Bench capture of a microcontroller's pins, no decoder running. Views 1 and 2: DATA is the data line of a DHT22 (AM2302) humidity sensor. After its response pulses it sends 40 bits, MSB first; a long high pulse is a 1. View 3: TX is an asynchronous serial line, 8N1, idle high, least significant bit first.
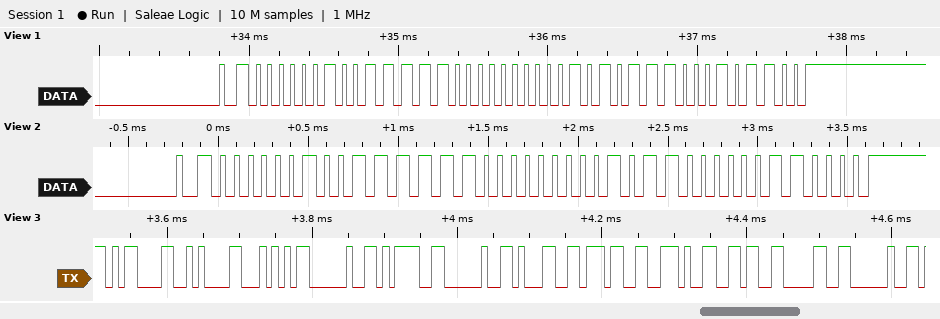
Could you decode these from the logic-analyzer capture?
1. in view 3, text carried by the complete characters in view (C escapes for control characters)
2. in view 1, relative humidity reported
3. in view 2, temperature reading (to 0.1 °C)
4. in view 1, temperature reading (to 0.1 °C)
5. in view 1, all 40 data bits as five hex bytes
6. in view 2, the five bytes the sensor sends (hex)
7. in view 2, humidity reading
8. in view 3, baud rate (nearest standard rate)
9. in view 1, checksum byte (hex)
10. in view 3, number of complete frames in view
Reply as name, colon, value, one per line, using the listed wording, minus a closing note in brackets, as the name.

in view 3, text carried by the complete characters in view: "\r\nT = 17.60 "
in view 1, relative humidity reported: 63.6 %
in view 2, temperature reading: 17.6 °C
in view 1, temperature reading: 17.4 °C
in view 1, all 40 data bits as five hex bytes: 02 7C 00 AE 2C
in view 2, the five bytes the sensor sends: 02 7E 00 B0 30
in view 2, humidity reading: 63.8 %
in view 3, baud rate: 115200 baud
in view 1, checksum byte: 0x2C
in view 3, number of complete frames in view: 12
